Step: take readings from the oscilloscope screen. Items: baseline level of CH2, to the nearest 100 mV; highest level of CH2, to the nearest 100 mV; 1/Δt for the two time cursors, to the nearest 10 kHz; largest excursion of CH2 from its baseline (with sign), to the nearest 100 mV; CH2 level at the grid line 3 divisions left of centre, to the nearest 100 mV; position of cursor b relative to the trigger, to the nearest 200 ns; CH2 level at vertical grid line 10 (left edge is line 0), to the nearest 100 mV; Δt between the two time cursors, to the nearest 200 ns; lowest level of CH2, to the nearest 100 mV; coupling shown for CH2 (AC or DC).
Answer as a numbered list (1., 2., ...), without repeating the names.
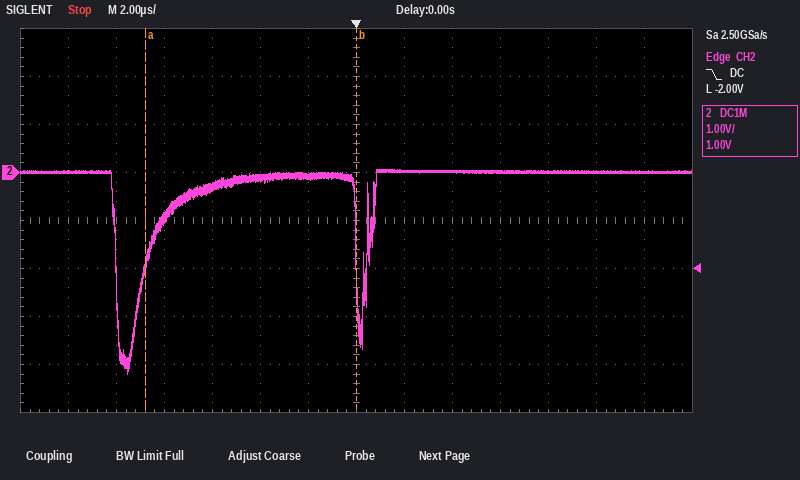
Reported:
1. 0.0 V
2. 100 mV
3. 110 kHz
4. -4.2 V
5. -300 mV
6. 0.0 µs
7. 0.0 V
8. 8.8 µs
9. -4.2 V
10. DC
